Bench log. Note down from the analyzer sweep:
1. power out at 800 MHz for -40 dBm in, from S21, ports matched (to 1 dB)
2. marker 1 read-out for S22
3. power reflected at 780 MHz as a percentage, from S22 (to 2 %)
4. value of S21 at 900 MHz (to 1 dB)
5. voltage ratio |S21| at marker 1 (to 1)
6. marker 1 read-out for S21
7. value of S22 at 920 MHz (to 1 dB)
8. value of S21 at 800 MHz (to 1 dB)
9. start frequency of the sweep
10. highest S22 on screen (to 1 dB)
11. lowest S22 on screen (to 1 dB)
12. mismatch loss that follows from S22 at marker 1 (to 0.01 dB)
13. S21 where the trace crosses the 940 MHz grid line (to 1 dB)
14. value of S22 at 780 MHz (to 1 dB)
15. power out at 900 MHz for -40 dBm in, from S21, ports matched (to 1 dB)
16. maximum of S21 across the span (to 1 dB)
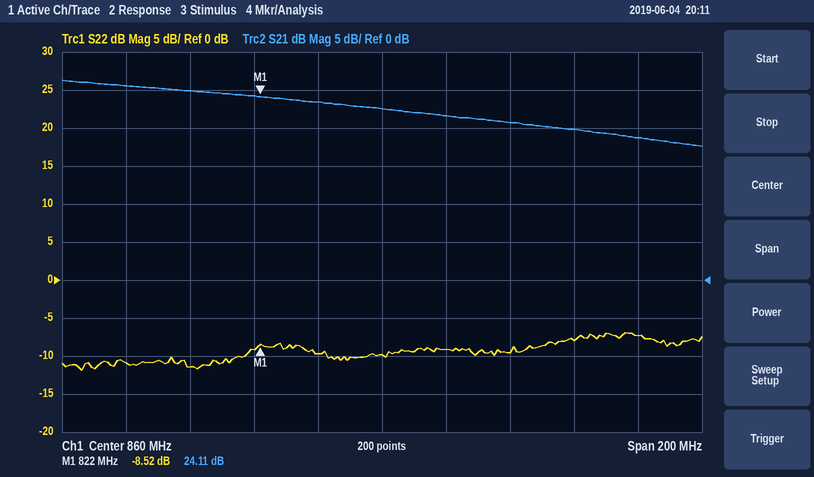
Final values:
-15 dBm
-8.52 dB
8 %
21 dB
16
24.11 dB
-8 dB
25 dB
760 MHz
-7 dB
-12 dB
0.66 dB
19 dB
-11 dB
-19 dBm
26 dB
